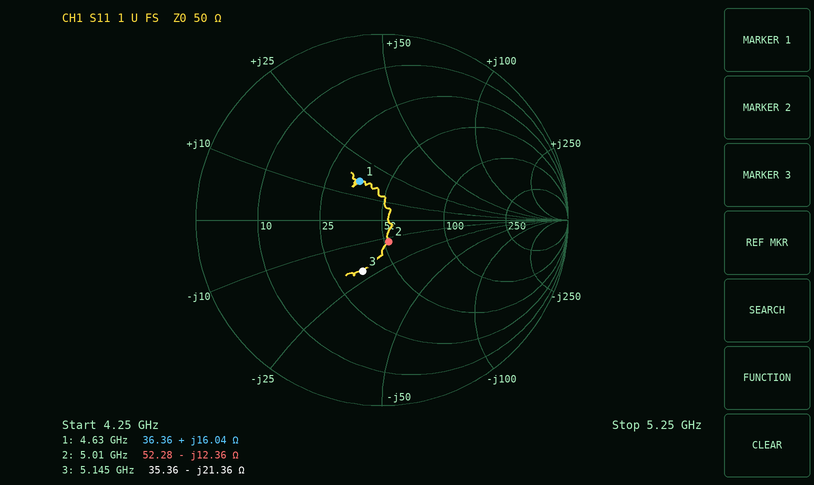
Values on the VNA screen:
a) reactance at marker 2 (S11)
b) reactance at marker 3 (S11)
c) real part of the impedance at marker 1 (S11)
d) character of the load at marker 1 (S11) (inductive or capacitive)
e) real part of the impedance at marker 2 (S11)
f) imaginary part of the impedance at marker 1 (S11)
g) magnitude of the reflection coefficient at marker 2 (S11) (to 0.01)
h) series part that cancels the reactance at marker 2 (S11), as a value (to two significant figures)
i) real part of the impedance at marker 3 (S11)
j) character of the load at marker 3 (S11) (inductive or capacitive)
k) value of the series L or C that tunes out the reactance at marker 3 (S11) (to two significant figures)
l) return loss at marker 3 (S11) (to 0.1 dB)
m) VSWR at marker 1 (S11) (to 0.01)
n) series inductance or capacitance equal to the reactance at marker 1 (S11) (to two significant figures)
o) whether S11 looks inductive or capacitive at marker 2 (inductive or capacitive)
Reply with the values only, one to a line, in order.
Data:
-12.36 Ω
-21.36 Ω
36.36 Ω
inductive
52.28 Ω
+16.04 Ω
0.12
390 pH
35.36 Ω
capacitive
660 pH
10.6 dB
1.63
550 pH
capacitive
